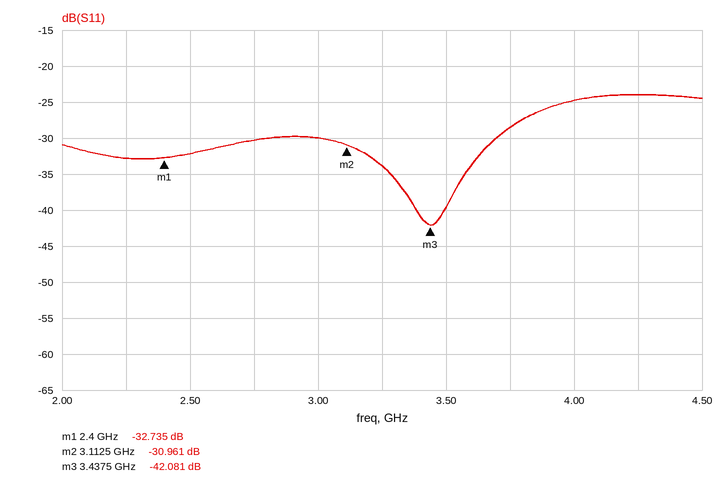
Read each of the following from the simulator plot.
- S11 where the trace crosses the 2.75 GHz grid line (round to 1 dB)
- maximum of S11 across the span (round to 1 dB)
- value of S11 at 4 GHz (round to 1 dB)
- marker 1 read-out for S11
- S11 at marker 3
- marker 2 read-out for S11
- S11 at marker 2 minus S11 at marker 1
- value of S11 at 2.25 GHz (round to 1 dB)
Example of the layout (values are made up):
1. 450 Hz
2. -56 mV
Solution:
1. -30 dB
2. -24 dB
3. -25 dB
4. -32.735 dB
5. -42.081 dB
6. -30.961 dB
7. 1.774 dB
8. -33 dB
